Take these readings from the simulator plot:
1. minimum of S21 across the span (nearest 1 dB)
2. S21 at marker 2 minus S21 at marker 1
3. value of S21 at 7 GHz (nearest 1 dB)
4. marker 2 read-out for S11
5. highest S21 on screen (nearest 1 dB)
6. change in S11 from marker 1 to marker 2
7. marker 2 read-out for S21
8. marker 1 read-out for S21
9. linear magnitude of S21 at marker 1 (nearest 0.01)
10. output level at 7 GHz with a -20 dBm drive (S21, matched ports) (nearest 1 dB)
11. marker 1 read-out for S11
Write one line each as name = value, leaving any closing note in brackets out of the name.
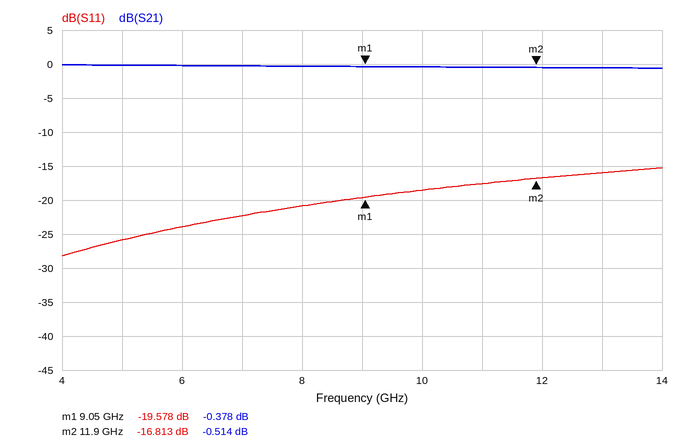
minimum of S21 across the span = -1 dB
S21 at marker 2 minus S21 at marker 1 = -0.136 dB
value of S21 at 7 GHz = 0 dB
marker 2 read-out for S11 = -16.813 dB
highest S21 on screen = 0 dB
change in S11 from marker 1 to marker 2 = 2.765 dB
marker 2 read-out for S21 = -0.514 dB
marker 1 read-out for S21 = -0.378 dB
linear magnitude of S21 at marker 1 = 0.96
output level at 7 GHz with a -20 dBm drive (S21, matched ports) = -20 dBm
marker 1 read-out for S11 = -19.578 dB
